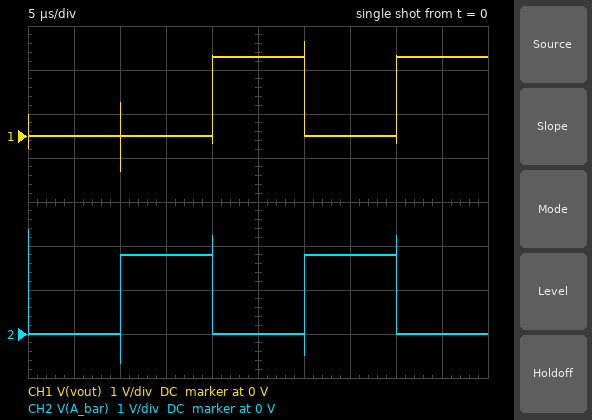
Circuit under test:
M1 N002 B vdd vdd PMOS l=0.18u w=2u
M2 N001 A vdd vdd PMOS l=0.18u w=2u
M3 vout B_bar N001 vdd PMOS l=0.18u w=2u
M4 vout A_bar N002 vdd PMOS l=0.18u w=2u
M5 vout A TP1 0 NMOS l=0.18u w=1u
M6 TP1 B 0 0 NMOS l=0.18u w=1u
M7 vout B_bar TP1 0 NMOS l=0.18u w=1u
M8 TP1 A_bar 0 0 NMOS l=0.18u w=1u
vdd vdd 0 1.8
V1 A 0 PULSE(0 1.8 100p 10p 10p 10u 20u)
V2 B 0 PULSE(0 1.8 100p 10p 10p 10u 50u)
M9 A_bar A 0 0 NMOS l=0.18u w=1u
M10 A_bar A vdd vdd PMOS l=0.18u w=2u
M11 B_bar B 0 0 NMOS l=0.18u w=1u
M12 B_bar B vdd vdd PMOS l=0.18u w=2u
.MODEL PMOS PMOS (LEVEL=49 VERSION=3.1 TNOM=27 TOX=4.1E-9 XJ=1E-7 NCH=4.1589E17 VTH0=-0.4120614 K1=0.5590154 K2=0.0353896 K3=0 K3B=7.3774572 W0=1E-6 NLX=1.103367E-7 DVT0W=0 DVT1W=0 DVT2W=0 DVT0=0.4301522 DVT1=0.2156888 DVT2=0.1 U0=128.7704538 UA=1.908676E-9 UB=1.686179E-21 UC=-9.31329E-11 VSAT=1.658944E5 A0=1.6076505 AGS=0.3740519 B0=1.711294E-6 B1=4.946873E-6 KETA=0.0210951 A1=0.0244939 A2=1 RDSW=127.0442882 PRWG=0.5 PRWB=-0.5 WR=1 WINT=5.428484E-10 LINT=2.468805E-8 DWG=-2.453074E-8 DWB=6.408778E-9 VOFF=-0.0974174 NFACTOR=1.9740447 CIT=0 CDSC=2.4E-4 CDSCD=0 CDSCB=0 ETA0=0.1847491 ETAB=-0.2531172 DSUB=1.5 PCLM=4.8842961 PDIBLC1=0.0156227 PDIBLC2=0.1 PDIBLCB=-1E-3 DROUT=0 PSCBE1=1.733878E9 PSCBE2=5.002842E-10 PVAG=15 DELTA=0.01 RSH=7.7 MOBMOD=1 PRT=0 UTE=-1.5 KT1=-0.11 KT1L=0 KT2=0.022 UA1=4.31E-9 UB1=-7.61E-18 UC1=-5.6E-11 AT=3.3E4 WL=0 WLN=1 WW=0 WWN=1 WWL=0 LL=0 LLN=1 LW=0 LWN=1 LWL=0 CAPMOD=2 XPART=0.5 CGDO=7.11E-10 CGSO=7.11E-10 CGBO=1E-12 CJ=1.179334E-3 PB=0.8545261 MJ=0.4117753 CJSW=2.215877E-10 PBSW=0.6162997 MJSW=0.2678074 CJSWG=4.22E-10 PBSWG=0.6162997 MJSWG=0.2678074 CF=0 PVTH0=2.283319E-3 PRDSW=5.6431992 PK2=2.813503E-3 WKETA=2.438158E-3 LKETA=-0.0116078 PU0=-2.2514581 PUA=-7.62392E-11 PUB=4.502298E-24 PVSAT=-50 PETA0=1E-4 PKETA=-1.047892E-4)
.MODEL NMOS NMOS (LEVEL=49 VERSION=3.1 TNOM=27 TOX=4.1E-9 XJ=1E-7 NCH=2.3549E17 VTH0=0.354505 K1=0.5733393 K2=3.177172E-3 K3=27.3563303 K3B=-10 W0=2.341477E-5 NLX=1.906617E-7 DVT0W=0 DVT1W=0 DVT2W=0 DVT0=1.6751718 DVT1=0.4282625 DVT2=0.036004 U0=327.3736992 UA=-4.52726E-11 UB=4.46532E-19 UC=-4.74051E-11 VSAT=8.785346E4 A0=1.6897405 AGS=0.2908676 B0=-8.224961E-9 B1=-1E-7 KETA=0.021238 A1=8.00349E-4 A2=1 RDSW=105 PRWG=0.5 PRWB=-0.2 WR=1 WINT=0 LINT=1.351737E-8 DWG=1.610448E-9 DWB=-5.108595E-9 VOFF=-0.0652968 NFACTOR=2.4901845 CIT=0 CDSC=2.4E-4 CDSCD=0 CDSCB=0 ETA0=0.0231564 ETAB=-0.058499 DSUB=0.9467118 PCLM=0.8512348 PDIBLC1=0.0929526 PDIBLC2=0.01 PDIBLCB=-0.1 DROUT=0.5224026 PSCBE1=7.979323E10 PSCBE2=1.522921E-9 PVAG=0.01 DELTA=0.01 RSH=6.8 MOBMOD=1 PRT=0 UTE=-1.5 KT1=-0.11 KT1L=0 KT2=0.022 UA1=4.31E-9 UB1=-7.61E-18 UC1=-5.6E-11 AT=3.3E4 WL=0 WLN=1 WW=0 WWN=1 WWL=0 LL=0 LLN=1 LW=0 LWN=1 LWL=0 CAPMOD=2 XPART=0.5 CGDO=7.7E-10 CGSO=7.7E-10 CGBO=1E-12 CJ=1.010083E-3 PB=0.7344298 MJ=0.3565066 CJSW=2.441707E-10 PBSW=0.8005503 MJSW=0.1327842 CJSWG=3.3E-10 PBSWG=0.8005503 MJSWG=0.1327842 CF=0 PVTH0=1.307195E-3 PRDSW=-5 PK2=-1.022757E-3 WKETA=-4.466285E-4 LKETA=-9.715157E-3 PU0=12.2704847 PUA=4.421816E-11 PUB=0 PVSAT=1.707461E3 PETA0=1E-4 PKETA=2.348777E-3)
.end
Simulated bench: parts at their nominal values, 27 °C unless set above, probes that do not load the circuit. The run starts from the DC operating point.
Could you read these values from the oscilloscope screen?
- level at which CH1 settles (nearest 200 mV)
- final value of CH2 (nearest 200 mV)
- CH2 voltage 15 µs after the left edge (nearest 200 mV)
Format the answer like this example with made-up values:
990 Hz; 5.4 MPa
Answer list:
1.8 V; 0 V; 1.8 V
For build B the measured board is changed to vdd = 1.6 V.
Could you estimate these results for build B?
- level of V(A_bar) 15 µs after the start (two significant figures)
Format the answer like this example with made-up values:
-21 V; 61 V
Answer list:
1.6 V
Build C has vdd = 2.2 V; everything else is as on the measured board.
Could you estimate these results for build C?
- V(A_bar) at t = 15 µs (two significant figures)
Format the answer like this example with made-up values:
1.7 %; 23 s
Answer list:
2.2 V
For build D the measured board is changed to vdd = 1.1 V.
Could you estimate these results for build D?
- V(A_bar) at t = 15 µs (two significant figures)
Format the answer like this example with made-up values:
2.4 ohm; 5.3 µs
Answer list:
1.1 V
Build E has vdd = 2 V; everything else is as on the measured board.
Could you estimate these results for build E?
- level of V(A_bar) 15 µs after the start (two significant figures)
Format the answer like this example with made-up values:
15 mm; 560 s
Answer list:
2.0 V
